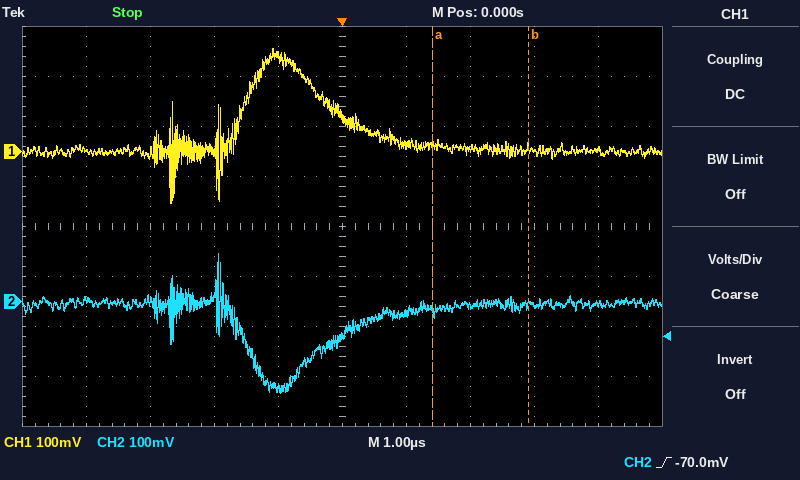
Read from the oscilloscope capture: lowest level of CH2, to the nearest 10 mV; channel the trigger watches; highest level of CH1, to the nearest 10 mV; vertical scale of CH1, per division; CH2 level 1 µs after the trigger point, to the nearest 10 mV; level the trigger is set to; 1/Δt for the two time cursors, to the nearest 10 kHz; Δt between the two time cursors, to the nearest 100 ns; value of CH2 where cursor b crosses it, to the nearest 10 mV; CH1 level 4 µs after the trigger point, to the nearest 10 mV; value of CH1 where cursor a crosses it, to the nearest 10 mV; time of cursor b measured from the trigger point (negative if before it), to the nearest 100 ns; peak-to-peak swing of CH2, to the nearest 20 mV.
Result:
-180 mV
CH2
210 mV
100 mV
-20 mV
-70.0 mV
670 kHz
1.5 µs
-10 mV
0 mV
10 mV
+2.9 µs
280 mV
